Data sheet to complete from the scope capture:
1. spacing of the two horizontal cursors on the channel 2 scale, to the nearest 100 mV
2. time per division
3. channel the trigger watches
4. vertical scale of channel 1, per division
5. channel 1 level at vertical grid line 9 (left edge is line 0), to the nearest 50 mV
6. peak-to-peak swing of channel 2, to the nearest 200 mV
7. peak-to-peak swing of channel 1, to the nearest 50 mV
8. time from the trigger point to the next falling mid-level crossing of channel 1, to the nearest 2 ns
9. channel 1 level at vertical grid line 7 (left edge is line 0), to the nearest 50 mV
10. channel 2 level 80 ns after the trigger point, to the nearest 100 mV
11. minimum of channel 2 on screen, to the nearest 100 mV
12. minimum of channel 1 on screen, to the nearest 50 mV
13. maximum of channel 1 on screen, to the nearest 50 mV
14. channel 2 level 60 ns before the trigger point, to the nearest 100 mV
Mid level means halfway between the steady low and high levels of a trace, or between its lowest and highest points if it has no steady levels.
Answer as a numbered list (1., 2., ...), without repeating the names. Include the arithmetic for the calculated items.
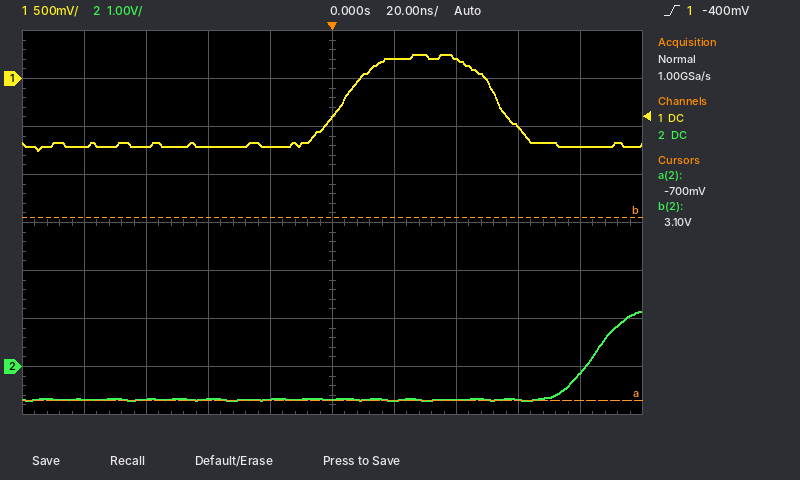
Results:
1. 3.8 V
2. 20 ns
3. channel 1
4. 500 mV
5. -700 mV
6. 1.8 V
7. 250 mV − (-750 mV) = 1.00 V
8. 54 ns
9. 200 mV
10. -100 mV
11. -700 mV
12. -750 mV
13. 250 mV
14. -700 mV
